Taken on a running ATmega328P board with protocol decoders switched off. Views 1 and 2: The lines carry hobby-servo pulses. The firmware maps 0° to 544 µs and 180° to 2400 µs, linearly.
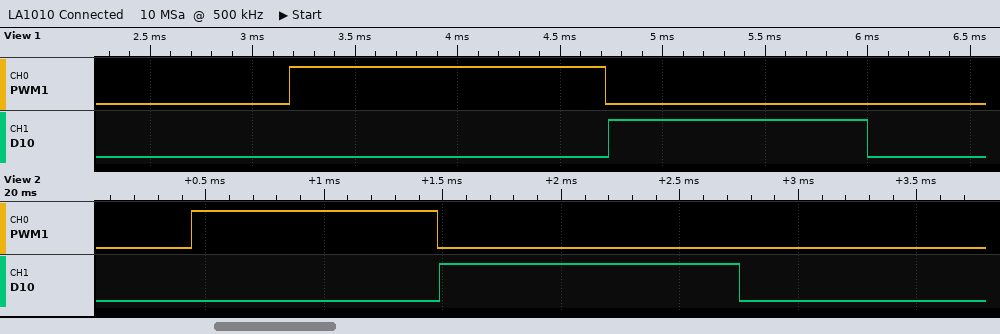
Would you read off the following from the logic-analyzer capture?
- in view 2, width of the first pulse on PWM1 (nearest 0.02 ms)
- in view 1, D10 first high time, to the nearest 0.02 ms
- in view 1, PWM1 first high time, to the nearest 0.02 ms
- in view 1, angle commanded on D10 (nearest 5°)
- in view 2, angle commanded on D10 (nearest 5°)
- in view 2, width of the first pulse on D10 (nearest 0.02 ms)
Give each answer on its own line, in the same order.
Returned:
1.04 ms
1.26 ms
1.54 ms
70°
70°
1.26 ms
